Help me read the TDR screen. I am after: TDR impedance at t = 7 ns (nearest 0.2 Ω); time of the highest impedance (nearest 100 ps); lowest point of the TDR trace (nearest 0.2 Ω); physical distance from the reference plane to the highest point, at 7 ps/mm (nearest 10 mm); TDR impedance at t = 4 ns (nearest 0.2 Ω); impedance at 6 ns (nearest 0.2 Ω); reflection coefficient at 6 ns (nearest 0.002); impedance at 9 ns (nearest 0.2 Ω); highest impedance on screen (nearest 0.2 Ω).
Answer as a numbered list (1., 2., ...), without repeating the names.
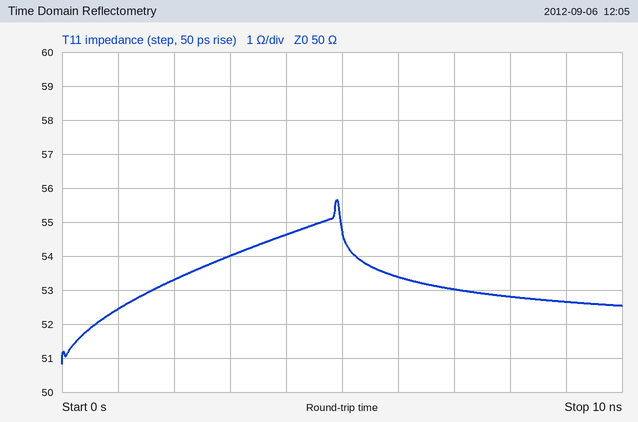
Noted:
1. 53.0 Ω
2. 4.9 ns
3. 50.8 Ω
4. 350 mm
5. 54.6 Ω
6. 53.4 Ω
7. +0.032
8. 52.6 Ω
9. 55.6 Ω
